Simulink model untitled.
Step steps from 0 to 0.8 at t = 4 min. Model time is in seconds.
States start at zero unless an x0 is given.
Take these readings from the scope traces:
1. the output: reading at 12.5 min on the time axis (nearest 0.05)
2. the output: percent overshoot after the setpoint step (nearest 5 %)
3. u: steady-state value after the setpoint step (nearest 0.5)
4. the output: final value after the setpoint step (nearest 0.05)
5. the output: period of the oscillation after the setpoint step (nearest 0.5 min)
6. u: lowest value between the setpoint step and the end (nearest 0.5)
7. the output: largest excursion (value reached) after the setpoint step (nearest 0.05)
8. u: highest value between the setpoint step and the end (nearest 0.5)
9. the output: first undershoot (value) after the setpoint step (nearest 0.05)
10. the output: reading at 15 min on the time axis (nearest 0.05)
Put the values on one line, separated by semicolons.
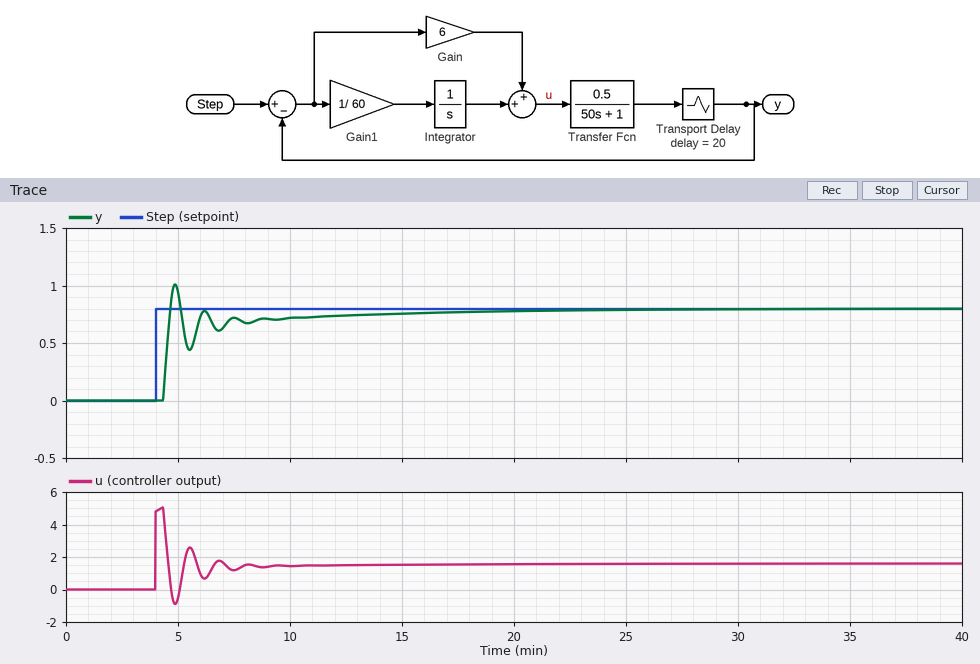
0.75; 25 %; 1.5; 0.80; 1.5 min; -1.0; 1.00; 5.0; 0.45; 0.75
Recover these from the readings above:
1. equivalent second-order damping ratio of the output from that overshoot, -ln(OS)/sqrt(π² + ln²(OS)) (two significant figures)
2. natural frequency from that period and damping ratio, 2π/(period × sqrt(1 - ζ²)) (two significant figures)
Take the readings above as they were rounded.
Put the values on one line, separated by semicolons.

0.40; 4.6 rad/min
